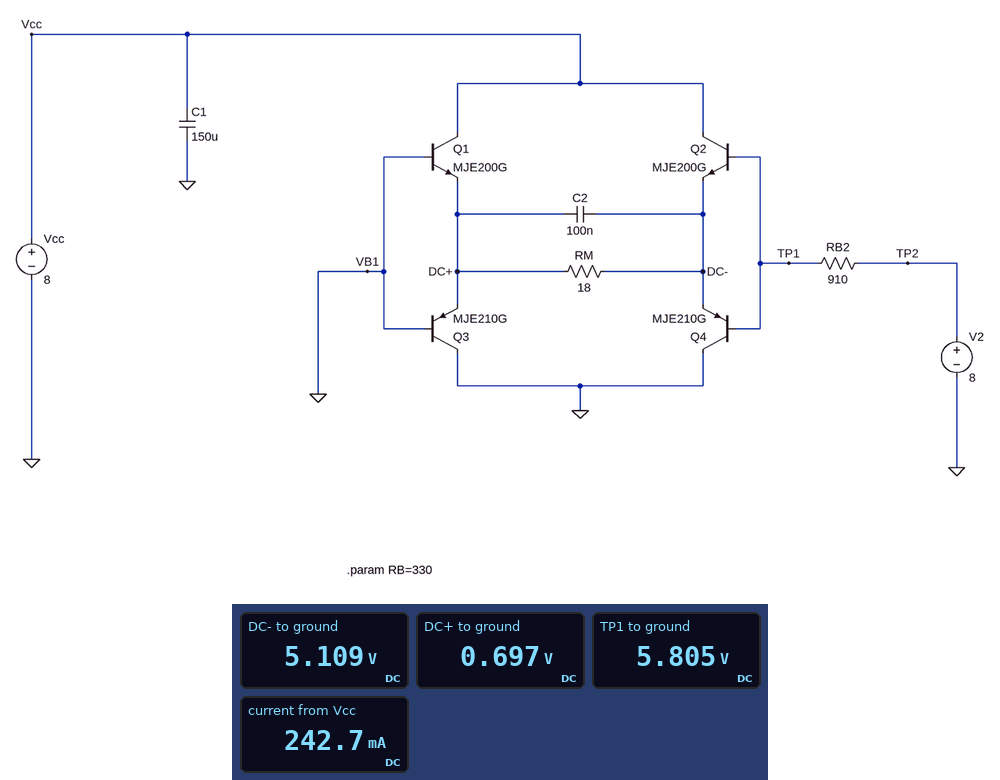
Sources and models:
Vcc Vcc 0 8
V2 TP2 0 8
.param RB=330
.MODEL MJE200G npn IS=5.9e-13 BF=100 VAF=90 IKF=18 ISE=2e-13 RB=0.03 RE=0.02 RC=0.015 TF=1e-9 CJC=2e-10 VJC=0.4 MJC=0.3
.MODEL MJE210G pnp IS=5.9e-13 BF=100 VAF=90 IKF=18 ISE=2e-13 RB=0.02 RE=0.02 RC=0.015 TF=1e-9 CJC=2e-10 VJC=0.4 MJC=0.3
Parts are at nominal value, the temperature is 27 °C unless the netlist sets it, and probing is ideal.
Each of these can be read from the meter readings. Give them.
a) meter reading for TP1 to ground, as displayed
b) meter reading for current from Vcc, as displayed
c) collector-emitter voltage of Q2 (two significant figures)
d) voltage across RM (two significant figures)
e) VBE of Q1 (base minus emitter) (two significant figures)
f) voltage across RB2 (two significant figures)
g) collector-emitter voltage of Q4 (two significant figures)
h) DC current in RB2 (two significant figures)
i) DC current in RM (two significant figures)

5.805 V
242.7 mA
2.9 V
4.4 V
-700 mV
2.2 V
-5.1 V
2.4 mA
250 mA
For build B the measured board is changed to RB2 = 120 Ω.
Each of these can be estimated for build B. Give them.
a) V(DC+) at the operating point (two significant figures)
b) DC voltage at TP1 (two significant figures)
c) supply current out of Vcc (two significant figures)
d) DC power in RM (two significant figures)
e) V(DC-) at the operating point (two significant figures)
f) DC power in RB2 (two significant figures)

710 mV
7.6 V
340 mA
2.1 W
6.9 V
1.4 mW
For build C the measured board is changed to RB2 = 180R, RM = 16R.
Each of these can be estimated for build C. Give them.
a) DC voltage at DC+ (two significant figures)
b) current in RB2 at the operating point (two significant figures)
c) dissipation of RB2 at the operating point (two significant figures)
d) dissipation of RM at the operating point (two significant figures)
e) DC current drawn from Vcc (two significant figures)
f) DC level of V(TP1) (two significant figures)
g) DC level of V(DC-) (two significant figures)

710 mV
3.7 mA
2.5 mW
2.2 W
370 mA
7.3 V
6.6 V
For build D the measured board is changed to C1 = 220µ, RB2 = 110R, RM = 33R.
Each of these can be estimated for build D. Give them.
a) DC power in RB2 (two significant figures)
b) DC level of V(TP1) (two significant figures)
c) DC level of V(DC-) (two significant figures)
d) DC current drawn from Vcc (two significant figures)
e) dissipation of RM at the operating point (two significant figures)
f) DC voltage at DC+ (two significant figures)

420 µW
7.8 V
7.1 V
190 mA
1.2 W
690 mV
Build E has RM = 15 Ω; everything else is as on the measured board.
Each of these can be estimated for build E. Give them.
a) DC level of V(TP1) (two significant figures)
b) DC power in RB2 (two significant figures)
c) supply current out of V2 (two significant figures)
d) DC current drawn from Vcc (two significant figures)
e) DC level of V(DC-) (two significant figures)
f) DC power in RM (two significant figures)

5.5 V
6.7 mW
2.7 mA
270 mA
4.8 V
1.1 W
